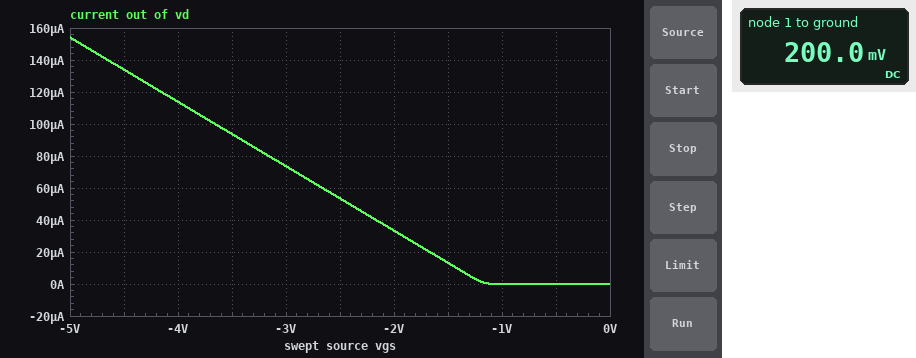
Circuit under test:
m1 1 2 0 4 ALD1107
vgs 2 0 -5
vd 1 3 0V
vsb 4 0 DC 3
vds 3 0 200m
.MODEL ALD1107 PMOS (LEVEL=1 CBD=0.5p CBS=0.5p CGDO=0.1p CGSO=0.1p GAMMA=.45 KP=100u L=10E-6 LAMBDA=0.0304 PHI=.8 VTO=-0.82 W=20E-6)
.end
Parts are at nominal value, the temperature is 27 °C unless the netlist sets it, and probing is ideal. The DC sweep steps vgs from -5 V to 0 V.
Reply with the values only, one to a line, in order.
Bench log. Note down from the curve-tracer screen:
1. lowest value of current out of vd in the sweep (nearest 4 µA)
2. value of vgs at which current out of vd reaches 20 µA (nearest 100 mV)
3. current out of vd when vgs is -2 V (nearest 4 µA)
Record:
0 A
-1.7 V
32 µA
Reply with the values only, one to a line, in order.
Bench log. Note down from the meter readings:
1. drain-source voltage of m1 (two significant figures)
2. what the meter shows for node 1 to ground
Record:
200 mV
200.0 mV
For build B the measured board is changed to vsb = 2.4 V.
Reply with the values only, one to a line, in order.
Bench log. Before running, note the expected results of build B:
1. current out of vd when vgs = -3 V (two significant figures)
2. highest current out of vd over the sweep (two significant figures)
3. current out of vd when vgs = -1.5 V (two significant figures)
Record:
77 µA
160 µA
16 µA
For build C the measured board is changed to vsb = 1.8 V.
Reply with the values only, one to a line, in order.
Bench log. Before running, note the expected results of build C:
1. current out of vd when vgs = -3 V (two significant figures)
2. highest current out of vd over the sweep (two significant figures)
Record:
80 µA
160 µA
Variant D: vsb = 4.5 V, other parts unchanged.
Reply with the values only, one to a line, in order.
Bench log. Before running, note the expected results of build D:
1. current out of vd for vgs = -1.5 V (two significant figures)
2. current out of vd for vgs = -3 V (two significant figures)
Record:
6.7 µA
67 µA
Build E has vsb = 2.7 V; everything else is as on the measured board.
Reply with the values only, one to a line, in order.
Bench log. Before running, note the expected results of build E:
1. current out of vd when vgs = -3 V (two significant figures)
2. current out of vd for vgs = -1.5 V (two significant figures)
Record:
75 µA
15 µA
